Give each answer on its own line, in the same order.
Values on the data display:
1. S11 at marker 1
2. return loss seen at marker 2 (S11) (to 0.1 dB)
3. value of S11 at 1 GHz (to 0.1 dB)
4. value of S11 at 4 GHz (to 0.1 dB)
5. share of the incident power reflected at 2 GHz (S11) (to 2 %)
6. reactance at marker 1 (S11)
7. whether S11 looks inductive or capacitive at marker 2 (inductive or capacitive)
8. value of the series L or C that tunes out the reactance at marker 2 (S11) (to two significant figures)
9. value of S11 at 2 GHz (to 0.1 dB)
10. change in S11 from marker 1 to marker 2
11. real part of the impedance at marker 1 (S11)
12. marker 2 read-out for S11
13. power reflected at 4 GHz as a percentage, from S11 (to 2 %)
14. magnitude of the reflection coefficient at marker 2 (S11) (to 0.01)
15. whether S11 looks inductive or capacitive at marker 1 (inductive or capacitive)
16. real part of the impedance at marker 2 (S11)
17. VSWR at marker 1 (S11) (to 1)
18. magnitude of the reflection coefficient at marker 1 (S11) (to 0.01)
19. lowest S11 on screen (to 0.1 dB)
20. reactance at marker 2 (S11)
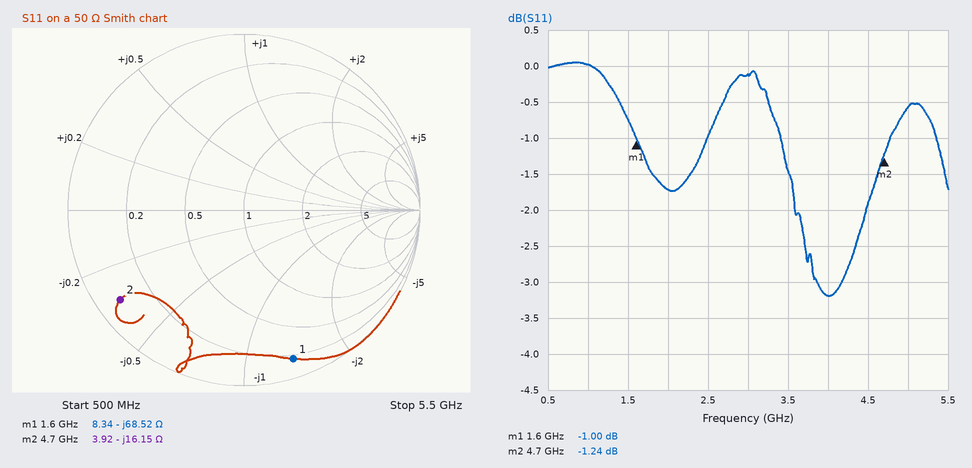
-1.00 dB
1.2 dB
0.0 dB
-3.2 dB
68 %
-68.52 Ω
capacitive
550 pH
-1.7 dB
-0.24 dB
8.34 Ω
-1.24 dB
48 %
0.87
capacitive
3.92 Ω
17
0.89
-3.2 dB
-16.15 Ω
